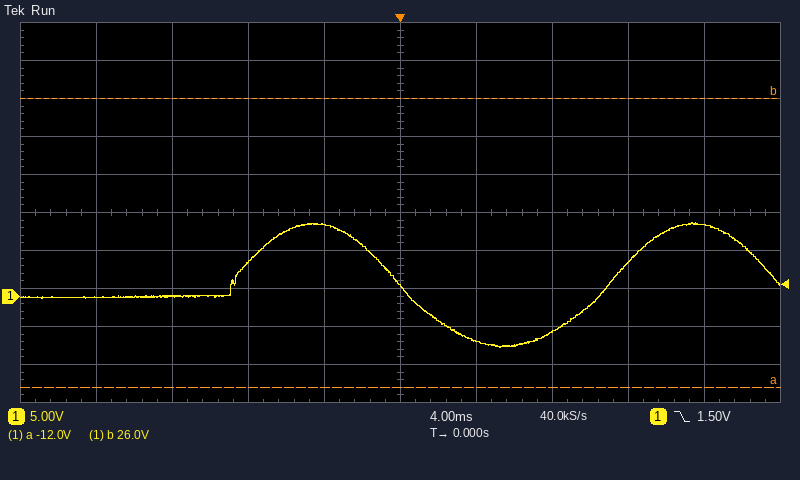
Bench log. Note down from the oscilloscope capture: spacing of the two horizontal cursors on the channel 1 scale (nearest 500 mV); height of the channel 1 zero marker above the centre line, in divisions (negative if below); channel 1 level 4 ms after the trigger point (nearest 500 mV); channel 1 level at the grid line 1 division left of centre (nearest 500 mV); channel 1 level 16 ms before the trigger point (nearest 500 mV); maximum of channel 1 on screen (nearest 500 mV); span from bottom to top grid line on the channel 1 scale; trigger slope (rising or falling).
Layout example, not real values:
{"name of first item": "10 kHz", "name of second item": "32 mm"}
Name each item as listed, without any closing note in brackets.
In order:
{"spacing of the two horizontal cursors on the channel 1 scale": "38.0 V", "height of the channel 1 zero marker above the centre line, in divisions": "-2.2 div", "channel 1 level 4 ms after the trigger point": "-6.0 V", "channel 1 level at the grid line 1 division left of centre": "9.5 V", "channel 1 level 16 ms before the trigger point": "0.0 V", "maximum of channel 1 on screen": "9.5 V", "span from bottom to top grid line on the channel 1 scale": "50 V", "trigger slope": "falling"}
